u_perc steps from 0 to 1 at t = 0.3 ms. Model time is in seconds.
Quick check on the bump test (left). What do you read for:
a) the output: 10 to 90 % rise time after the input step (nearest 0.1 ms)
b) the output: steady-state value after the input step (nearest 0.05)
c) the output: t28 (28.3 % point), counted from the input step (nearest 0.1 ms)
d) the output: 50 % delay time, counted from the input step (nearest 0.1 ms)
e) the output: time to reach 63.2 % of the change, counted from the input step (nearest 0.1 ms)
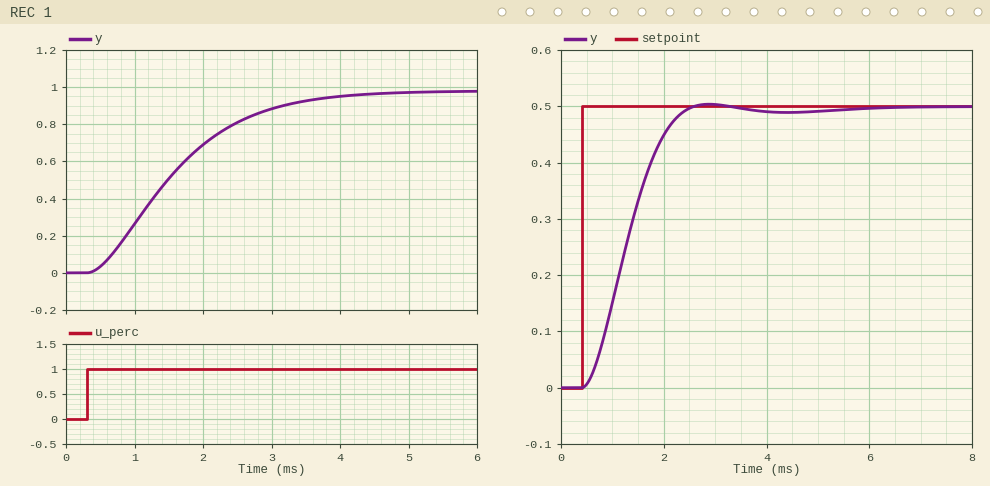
2.3 ms
1.00
0.7 ms
1.2 ms
1.5 ms
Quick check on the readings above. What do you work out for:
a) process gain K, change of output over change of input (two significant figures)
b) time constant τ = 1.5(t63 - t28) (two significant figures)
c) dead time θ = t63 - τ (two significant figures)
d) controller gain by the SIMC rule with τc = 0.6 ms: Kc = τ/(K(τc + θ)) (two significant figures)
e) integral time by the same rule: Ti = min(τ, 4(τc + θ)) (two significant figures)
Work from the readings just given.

1.0
1.2 ms
0.30 ms
1.3
1.2 ms
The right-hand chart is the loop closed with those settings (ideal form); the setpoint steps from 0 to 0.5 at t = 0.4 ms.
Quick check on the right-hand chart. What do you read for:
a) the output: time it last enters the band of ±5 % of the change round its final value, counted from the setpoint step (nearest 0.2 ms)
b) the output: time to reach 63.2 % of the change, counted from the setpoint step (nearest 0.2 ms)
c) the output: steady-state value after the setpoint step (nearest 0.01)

1.8 ms
1.0 ms
0.50
